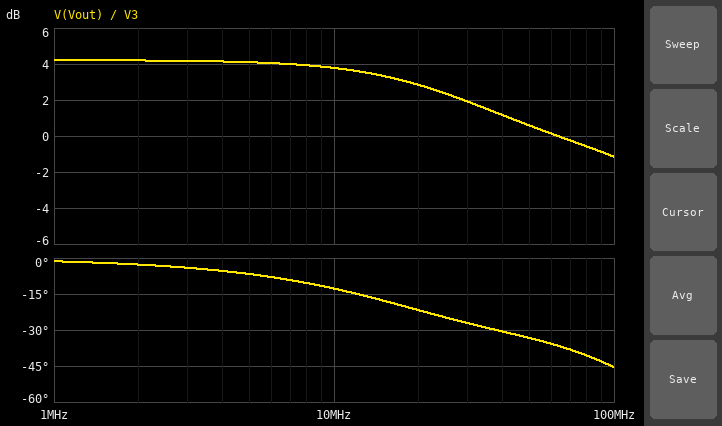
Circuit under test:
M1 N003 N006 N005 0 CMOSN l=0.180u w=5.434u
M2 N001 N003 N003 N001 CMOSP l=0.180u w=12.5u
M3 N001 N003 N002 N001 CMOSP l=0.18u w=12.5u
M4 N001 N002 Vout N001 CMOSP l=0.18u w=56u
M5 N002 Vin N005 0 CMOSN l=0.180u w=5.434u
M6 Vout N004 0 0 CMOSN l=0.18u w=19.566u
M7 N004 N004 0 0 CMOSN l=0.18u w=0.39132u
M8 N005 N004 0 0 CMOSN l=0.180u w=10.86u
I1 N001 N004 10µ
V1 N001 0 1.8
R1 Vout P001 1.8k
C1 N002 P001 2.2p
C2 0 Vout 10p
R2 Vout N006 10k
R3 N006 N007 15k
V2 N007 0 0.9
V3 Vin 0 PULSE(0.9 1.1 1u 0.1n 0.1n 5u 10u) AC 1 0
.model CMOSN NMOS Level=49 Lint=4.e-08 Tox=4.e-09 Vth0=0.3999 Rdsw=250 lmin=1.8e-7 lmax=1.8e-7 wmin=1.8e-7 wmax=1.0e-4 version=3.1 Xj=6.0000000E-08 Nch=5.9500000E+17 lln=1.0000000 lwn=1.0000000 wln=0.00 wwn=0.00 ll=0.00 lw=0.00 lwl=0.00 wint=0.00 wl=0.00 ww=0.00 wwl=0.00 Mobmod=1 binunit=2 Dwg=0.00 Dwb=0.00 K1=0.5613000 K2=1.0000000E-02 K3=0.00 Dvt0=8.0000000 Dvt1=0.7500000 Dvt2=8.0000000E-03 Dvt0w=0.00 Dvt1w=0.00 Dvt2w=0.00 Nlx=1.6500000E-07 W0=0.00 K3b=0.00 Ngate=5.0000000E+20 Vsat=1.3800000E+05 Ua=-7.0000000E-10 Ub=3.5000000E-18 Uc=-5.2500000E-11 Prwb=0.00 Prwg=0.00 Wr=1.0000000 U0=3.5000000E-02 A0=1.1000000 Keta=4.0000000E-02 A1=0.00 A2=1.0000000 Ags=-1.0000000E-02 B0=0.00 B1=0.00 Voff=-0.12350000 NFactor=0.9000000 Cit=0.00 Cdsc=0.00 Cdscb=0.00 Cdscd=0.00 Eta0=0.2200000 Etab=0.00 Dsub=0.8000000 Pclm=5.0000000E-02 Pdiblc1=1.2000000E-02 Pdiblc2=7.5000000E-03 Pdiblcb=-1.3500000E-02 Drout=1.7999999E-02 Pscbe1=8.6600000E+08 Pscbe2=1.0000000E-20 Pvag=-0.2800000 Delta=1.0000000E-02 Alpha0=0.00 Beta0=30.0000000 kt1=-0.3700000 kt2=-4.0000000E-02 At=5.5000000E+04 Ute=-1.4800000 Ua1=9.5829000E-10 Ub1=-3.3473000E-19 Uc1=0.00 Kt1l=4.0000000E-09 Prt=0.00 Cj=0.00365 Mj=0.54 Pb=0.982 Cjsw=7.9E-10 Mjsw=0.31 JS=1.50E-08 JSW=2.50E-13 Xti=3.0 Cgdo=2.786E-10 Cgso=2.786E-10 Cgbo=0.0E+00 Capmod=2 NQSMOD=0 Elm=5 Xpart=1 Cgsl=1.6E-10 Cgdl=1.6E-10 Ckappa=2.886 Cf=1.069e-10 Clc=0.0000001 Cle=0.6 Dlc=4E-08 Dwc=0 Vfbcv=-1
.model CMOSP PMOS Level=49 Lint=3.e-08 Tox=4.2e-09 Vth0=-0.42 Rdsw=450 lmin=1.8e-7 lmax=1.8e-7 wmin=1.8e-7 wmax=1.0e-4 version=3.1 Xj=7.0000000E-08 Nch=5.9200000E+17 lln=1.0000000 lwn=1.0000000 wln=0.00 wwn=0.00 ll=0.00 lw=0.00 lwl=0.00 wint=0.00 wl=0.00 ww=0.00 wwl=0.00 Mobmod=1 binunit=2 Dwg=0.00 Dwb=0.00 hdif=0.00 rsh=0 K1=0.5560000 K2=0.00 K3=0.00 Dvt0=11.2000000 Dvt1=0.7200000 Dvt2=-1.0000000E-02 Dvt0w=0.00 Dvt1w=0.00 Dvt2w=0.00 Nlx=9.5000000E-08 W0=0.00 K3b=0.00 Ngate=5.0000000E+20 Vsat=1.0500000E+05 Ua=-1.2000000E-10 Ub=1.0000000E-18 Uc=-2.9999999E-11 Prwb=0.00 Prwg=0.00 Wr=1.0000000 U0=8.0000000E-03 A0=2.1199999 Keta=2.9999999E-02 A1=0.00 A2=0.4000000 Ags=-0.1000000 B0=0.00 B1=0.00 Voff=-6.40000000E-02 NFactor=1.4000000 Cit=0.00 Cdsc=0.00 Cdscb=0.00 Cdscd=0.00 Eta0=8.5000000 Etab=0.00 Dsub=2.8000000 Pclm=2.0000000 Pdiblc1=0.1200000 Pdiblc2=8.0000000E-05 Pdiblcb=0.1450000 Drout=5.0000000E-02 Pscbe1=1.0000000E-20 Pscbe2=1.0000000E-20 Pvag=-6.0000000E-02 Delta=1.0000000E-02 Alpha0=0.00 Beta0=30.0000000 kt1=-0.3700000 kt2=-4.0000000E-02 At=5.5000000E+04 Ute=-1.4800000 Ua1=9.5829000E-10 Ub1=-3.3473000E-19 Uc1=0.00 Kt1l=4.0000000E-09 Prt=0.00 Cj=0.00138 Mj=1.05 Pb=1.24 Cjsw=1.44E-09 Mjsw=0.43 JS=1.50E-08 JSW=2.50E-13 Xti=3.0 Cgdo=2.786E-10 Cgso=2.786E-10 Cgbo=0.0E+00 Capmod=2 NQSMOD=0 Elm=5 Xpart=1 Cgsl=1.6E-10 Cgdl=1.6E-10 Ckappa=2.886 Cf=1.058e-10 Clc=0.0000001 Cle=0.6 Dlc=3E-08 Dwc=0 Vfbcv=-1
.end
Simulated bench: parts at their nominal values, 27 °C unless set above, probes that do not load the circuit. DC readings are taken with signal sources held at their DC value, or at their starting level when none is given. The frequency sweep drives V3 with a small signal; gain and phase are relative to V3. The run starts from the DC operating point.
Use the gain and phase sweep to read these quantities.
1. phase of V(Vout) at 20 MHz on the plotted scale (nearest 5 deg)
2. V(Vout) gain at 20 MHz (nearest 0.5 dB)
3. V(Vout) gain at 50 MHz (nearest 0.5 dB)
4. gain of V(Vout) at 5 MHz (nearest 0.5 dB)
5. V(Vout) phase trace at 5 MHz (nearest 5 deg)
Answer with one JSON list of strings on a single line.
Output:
["-20 deg", "3.0 dB", "0.5 dB", "4.0 dB", "-5 deg"]
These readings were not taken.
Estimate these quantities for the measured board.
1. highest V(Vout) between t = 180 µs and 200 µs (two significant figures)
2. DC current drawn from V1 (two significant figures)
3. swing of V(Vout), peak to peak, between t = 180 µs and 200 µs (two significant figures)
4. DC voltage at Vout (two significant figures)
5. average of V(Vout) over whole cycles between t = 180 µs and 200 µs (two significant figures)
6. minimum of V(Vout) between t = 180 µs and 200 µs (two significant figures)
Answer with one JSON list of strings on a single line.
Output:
["1.2 V", "920 µA", "320 mV", "900 mV", "1.1 V", "900 mV"]
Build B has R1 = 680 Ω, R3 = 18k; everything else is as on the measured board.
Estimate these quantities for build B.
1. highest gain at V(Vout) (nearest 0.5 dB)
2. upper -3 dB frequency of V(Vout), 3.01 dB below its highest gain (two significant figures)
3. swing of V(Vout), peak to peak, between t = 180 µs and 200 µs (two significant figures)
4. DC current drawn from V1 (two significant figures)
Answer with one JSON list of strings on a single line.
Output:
["3.5 dB", "49 MHz", "300 mV", "920 µA"]
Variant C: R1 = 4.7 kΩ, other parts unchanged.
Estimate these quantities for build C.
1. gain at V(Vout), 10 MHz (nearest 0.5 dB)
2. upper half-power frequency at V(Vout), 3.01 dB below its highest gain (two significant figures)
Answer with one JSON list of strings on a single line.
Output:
["3.5 dB", "240 MHz"]
